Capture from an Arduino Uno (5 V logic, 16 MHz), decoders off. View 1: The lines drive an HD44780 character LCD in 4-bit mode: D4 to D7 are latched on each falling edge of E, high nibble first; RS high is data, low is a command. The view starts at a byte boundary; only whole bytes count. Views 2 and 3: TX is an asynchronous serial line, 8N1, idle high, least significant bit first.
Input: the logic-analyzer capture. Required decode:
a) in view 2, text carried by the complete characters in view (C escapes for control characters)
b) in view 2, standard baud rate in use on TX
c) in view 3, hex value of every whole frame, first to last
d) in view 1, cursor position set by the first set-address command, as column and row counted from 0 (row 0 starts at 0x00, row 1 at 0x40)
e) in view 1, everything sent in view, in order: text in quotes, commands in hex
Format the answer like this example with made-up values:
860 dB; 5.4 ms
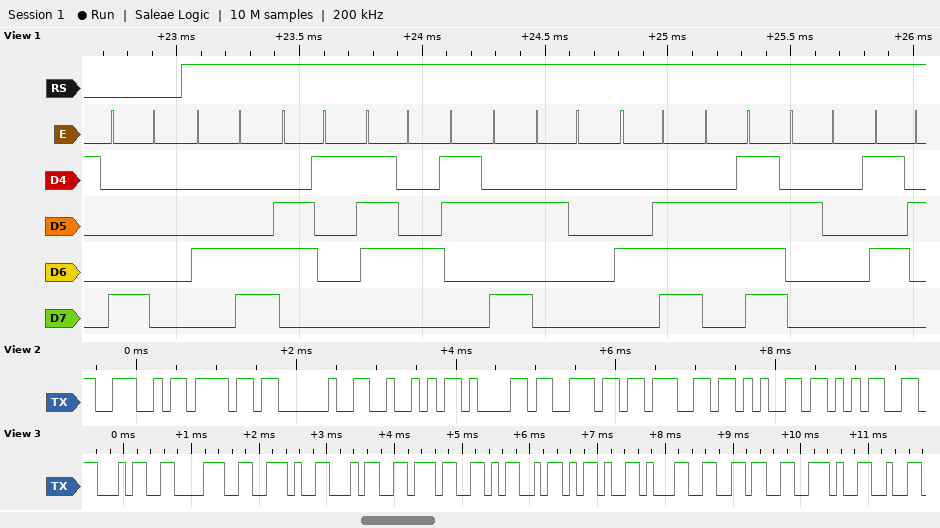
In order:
"No Range5"; 9600 baud; 34 38 2E 34 37 4D 2D 31 36 2E; column 0, row 0; 0x80 "Lat: No R"
